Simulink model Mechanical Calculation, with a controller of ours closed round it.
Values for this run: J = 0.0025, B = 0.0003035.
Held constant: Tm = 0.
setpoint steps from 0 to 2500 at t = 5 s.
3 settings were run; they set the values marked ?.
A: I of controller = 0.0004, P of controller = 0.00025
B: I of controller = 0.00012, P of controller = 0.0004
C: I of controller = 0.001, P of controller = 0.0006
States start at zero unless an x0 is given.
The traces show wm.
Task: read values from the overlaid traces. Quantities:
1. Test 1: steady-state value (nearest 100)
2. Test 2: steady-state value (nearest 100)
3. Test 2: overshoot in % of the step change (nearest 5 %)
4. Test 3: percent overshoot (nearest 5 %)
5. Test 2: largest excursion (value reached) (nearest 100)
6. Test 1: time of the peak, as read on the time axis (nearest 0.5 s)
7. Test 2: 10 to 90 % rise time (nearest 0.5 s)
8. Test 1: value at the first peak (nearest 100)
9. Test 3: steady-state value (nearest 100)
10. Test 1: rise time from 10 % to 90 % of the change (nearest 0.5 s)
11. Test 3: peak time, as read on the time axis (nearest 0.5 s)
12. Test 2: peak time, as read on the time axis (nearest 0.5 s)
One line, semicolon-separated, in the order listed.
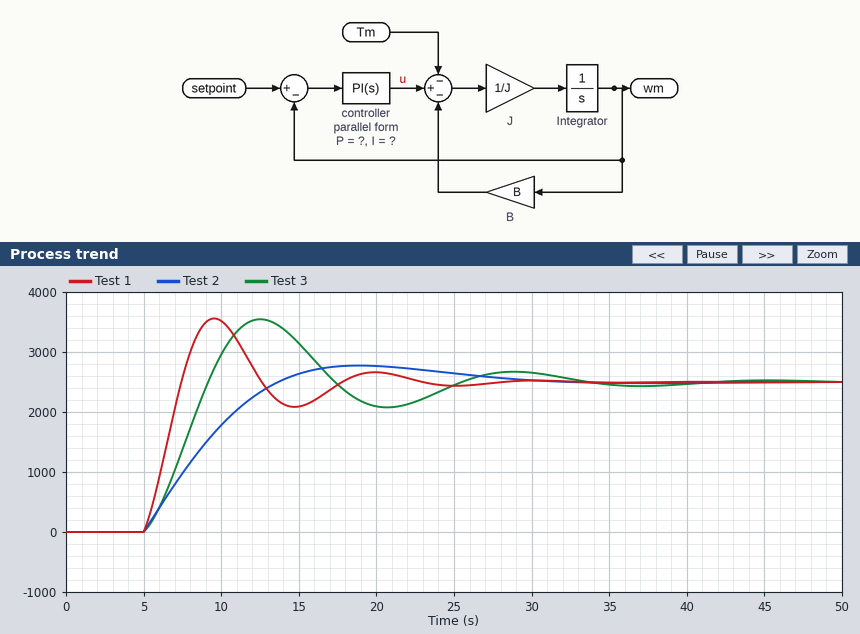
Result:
2500; 2500; 10 %; 40 %; 2800; 9.5 s; 6.5 s; 3600; 2500; 2.0 s; 12.5 s; 19.0 s
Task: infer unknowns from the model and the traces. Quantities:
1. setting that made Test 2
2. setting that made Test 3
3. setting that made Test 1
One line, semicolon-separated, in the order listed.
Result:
B; A; C
